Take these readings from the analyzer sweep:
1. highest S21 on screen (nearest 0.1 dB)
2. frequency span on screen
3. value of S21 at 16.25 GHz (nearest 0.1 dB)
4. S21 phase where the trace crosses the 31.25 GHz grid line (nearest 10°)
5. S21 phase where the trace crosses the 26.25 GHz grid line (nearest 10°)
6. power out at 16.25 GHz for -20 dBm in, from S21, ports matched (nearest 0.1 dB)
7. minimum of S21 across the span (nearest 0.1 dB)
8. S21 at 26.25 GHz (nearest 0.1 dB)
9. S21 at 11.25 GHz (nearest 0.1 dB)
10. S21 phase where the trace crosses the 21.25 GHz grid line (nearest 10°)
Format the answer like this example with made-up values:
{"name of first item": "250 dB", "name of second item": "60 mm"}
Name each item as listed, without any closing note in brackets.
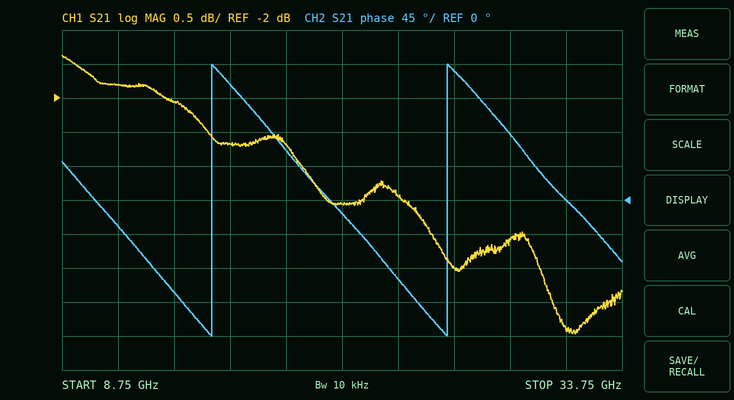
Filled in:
{"highest S21 on screen": "-1.4 dB", "frequency span on screen": "25 GHz", "value of S21 at 16.25 GHz": "-2.7 dB", "S21 phase where the trace crosses the 31.25 GHz grid line": "0°", "S21 phase where the trace crosses the 26.25 GHz grid line": "170°", "power out at 16.25 GHz for -20 dBm in, from S21, ports matched": "-22.7 dBm", "minimum of S21 across the span": "-5.5 dB", "S21 at 26.25 GHz": "-4.5 dB", "S21 at 11.25 GHz": "-1.8 dB", "S21 phase where the trace crosses the 21.25 GHz grid line": "-20°"}
